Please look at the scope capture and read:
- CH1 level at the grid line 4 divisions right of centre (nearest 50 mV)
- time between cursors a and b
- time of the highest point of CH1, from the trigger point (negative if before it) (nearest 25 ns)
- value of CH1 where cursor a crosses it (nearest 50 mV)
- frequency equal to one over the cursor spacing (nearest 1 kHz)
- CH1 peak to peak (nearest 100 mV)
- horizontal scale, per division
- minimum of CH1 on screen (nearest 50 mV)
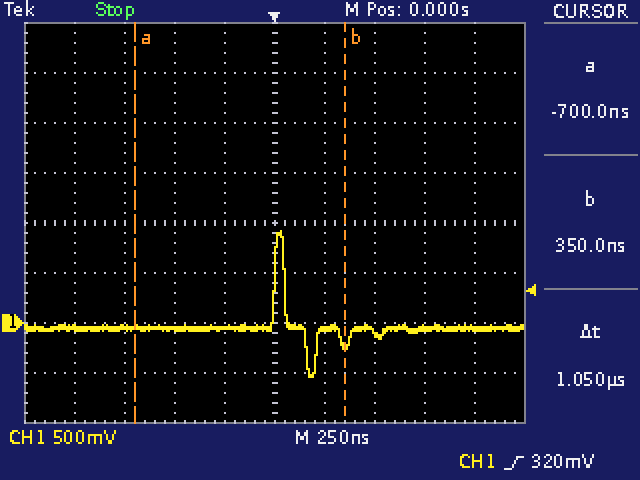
-50 mV
1.05 µs
+25 ns
-50 mV
952 kHz
1.50 V
250 ns
-550 mV
